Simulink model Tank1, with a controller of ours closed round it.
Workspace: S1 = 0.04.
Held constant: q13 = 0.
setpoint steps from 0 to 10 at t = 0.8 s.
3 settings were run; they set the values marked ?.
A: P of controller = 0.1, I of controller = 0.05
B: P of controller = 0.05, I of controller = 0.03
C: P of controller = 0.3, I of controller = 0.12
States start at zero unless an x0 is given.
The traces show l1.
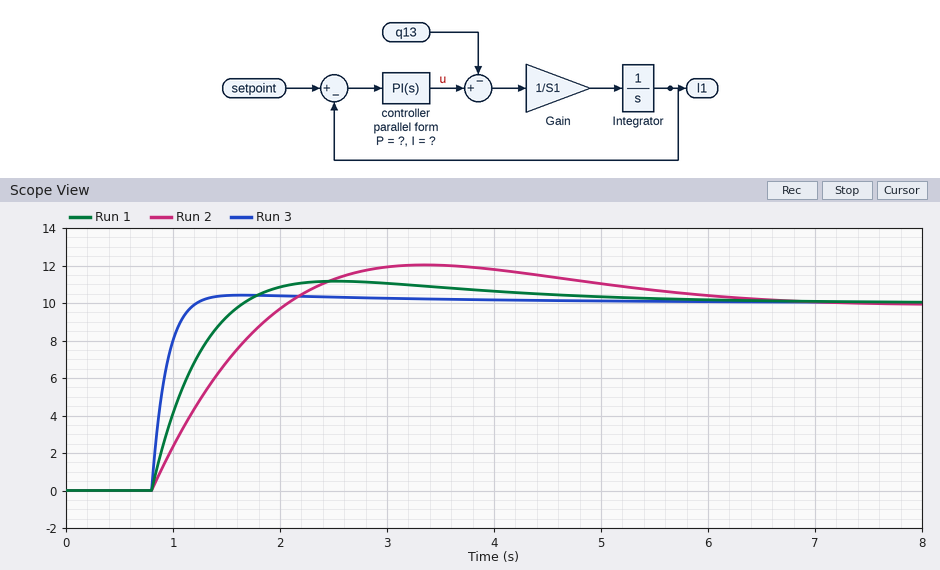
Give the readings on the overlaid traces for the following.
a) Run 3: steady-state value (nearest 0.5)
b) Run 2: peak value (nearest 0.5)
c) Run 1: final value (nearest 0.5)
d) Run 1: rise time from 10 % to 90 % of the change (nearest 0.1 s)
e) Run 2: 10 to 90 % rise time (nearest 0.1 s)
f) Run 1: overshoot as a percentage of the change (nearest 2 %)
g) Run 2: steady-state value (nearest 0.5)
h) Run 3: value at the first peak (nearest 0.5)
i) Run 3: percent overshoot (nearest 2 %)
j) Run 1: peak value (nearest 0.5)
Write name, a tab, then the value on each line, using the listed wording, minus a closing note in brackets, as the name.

Run 3: steady-state value	10.0
Run 2: peak value	12.0
Run 1: final value	10.0
Run 1: rise time from 10 % to 90 % of the change	0.6 s
Run 2: 10 to 90 % rise time	1.0 s
Run 1: overshoot as a percentage of the change	12 %
Run 2: steady-state value	10.0
Run 3: value at the first peak	10.5
Run 3: percent overshoot	4 %
Run 1: peak value	11.0
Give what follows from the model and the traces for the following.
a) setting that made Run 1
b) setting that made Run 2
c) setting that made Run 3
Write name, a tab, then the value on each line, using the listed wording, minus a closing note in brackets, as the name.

setting that made Run 1	A
setting that made Run 2	B
setting that made Run 3	C
